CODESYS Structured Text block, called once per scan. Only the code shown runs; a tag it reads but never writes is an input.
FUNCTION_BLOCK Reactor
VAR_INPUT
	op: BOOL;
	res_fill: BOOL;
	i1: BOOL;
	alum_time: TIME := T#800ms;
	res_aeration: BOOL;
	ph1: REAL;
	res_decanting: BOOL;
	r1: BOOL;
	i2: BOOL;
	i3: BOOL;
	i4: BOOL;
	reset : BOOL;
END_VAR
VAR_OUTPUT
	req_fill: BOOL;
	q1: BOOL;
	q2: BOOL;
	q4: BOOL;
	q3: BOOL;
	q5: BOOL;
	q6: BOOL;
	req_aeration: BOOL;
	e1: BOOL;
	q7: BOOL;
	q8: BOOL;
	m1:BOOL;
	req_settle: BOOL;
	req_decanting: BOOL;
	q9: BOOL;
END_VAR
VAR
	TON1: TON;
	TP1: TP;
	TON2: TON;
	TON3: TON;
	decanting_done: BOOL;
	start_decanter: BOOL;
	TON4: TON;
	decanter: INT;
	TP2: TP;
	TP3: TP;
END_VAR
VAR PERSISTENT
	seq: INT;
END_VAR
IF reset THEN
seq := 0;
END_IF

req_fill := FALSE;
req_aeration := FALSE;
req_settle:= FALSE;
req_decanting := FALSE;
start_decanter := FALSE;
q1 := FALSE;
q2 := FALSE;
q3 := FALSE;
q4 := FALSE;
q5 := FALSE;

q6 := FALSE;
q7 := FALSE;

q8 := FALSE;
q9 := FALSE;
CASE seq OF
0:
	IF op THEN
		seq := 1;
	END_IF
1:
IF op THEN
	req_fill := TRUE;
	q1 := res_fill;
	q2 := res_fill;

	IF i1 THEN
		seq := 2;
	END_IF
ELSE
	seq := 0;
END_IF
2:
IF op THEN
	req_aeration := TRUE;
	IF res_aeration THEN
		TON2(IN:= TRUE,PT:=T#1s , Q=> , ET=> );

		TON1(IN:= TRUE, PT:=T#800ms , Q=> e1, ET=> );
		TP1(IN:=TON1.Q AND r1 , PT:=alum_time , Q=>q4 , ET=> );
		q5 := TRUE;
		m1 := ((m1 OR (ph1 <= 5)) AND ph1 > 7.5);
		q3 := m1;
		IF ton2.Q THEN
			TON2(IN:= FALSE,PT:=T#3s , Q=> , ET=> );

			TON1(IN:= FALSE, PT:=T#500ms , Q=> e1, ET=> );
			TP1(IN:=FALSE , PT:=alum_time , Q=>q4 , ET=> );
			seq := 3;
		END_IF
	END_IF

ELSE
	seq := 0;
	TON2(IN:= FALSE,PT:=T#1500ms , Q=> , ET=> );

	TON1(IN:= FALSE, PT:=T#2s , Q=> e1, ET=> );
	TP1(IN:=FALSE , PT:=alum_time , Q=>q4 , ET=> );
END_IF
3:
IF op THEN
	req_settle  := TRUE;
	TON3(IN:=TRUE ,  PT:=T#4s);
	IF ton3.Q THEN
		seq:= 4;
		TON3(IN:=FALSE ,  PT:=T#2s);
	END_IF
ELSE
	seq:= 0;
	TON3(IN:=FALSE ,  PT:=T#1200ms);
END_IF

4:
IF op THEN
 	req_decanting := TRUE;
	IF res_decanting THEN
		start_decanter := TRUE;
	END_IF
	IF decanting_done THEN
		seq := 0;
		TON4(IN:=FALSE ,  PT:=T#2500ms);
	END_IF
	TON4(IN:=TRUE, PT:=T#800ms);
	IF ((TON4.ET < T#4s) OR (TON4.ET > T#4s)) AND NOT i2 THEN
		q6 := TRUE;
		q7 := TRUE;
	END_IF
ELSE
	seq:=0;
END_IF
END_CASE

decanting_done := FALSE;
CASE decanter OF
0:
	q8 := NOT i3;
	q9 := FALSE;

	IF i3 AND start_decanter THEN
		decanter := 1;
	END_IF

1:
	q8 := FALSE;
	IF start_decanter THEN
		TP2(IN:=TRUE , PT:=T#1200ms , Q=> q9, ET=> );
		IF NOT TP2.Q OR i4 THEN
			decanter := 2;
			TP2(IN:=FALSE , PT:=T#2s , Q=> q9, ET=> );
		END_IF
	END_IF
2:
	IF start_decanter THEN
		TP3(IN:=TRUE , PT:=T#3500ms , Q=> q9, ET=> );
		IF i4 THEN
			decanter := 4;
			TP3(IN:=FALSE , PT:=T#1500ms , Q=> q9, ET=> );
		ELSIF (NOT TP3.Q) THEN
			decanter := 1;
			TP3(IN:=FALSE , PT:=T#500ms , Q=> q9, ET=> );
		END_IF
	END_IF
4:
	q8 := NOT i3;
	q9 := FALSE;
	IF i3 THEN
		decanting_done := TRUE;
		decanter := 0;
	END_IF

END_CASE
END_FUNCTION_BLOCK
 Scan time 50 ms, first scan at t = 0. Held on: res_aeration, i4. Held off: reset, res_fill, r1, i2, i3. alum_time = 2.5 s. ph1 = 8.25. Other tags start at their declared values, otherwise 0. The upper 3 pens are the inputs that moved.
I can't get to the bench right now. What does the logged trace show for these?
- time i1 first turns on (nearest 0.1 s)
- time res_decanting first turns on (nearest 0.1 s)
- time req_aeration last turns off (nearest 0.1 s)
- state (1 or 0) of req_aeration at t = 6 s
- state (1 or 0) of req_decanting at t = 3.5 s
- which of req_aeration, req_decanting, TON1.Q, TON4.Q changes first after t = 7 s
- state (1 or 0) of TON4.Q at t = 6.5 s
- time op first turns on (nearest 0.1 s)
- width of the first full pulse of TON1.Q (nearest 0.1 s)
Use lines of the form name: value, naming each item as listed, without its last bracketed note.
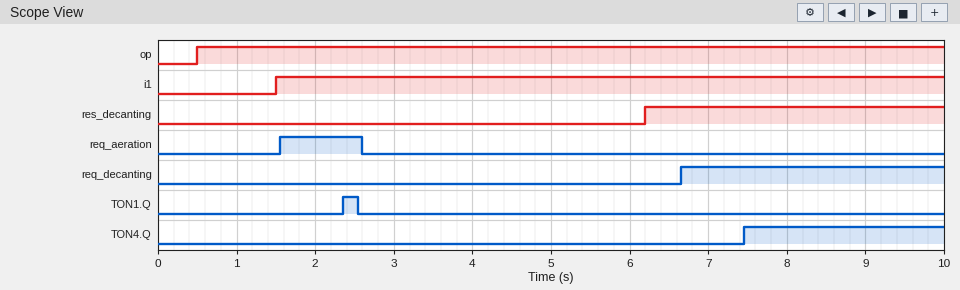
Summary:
time i1 first turns on: 1.5 s
time res_decanting first turns on: 6.2 s
time req_aeration last turns off: 2.6 s
state (1 or 0) of req_aeration at t = 6 s: 0
state (1 or 0) of req_decanting at t = 3.5 s: 0
which of req_aeration, req_decanting, TON1.Q, TON4.Q changes first after t = 7 s: TON4.Q
state (1 or 0) of TON4.Q at t = 6.5 s: 0
time op first turns on: 0.5 s
width of the first full pulse of TON1.Q: 0.2 s
